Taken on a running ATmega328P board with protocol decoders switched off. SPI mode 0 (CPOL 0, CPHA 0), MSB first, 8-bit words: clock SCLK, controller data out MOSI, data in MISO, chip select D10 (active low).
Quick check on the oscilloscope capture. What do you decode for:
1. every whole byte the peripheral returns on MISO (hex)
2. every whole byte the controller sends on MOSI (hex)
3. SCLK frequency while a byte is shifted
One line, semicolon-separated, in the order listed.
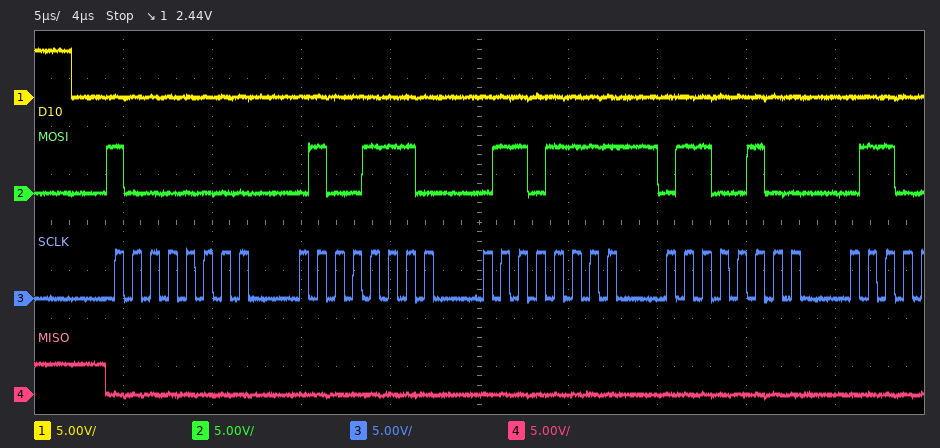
00 00 00 00; 80 4E 6F 64; 1 MHz
